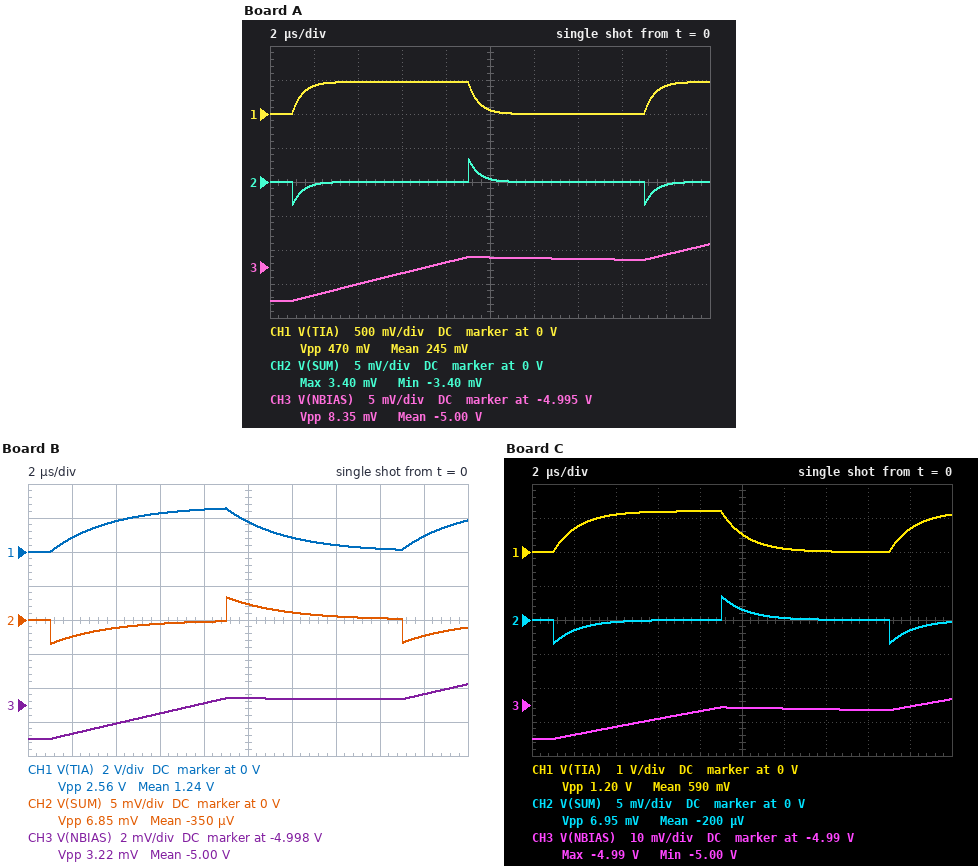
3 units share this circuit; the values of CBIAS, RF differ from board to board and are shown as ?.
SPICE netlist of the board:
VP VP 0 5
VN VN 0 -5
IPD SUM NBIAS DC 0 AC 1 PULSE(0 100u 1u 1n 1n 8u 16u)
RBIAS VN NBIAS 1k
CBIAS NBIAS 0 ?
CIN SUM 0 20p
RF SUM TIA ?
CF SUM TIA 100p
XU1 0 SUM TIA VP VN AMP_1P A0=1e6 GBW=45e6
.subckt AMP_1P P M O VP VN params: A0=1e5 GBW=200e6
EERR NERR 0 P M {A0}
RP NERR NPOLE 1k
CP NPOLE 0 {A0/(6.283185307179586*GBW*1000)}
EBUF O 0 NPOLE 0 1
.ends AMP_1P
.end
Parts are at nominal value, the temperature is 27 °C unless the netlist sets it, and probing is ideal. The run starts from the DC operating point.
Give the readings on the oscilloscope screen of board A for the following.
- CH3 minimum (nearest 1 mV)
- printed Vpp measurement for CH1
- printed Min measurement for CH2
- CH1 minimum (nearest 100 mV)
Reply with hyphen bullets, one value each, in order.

- -5.000 V
- 470 mV
- -3.40 mV
- 0 V
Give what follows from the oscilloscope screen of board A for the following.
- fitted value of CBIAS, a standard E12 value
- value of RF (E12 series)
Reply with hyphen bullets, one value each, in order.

- 120 nF
- 4.7 kΩ
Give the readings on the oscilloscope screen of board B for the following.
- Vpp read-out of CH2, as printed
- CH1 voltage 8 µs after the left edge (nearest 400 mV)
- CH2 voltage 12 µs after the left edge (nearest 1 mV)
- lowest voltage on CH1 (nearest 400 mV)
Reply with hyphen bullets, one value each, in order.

- 6.85 mV
- 2.4 V
- 1 mV
- 0 V
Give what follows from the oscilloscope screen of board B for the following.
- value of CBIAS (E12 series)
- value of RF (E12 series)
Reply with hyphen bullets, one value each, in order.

- 330 nF
- 27 kΩ
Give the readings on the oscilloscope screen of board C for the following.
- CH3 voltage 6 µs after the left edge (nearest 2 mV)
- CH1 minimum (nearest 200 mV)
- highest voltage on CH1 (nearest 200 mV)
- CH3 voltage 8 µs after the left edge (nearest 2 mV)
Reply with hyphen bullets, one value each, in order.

- -4.994 V
- 0 V
- 1.2 V
- -4.992 V
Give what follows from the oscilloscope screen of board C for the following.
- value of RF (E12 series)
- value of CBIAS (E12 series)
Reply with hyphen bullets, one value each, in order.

- 12 kΩ
- 82 nF
